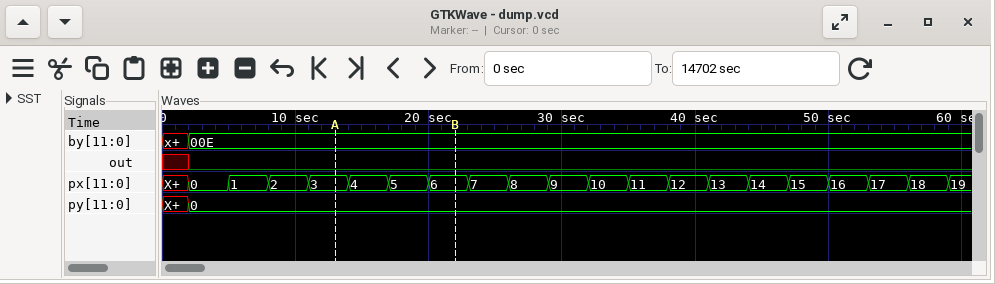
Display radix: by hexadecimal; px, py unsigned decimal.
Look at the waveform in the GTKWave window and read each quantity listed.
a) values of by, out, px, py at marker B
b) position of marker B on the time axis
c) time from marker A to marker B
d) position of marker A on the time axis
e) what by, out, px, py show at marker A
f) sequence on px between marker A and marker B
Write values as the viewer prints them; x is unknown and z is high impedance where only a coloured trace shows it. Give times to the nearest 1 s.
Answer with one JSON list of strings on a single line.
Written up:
["by=00E, out=0, px=6, py=0", "22 s", "9 s", "13 s", "by=00E, out=0, px=3, py=0", "3, 4, 5, 6"]
